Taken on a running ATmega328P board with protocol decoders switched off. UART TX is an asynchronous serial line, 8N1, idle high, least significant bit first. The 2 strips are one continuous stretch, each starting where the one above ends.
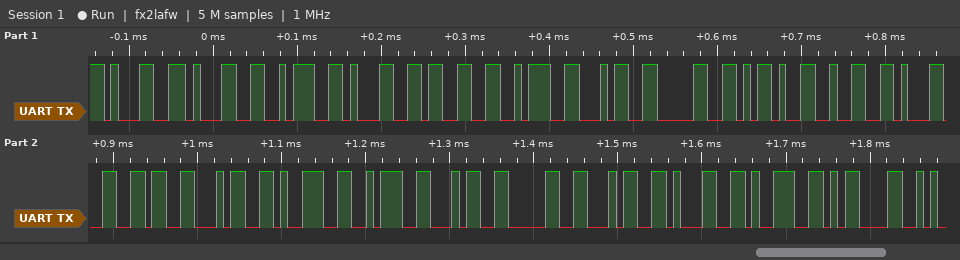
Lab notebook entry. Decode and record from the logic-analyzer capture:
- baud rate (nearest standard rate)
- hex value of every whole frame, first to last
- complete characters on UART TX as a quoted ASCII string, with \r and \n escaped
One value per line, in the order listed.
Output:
115200 baud
0x31 0x31 0x3A 0x31 0x33 0x3A 0x34 0x30 0x2D 0x32 0x31 0x36 0x34 0x39 0x3A 0x34 0x30 0x34 0x31 0x39 0x0D
"11:13:40-21649:40419\r"
